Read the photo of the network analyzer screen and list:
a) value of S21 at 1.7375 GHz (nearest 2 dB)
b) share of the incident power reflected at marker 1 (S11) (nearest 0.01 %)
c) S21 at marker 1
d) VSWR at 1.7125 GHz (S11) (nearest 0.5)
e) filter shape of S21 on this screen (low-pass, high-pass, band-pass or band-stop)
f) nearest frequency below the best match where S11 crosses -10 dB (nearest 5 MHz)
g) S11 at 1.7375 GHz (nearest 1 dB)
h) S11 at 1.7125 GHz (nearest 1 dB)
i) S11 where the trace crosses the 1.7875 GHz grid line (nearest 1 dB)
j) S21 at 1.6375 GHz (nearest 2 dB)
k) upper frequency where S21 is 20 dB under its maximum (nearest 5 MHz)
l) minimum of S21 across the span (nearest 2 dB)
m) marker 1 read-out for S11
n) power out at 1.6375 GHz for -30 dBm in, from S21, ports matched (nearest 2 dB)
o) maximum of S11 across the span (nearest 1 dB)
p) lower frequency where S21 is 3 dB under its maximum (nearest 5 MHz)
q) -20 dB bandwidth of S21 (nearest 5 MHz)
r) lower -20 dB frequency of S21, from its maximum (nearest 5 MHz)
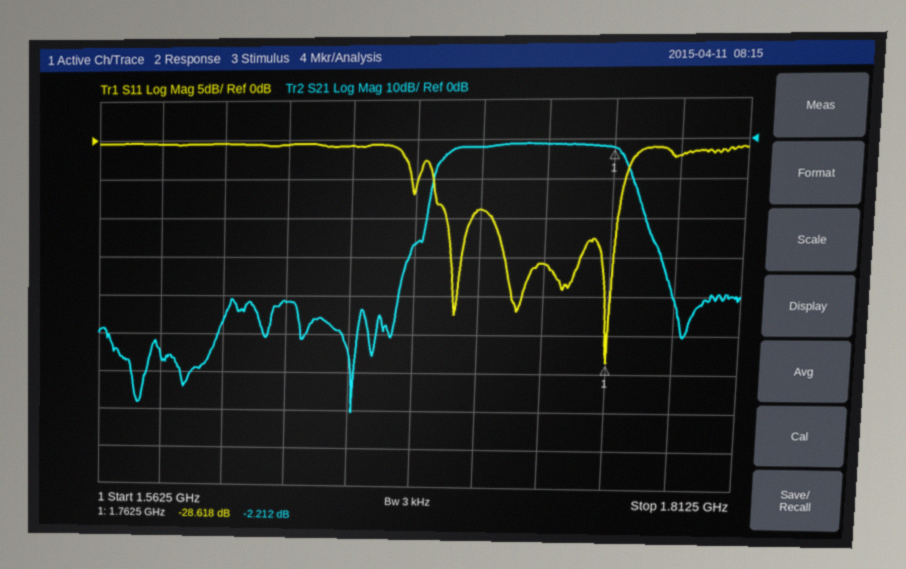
-2 dB
0.14 %
-2.212 dB
2.0
band-pass
1.715 GHz
-16 dB
-9 dB
-2 dB
-42 dB
1.775 GHz
-70 dB
-28.618 dB
-72 dBm
0 dB
1.700 GHz
85 MHz
1.690 GHz
